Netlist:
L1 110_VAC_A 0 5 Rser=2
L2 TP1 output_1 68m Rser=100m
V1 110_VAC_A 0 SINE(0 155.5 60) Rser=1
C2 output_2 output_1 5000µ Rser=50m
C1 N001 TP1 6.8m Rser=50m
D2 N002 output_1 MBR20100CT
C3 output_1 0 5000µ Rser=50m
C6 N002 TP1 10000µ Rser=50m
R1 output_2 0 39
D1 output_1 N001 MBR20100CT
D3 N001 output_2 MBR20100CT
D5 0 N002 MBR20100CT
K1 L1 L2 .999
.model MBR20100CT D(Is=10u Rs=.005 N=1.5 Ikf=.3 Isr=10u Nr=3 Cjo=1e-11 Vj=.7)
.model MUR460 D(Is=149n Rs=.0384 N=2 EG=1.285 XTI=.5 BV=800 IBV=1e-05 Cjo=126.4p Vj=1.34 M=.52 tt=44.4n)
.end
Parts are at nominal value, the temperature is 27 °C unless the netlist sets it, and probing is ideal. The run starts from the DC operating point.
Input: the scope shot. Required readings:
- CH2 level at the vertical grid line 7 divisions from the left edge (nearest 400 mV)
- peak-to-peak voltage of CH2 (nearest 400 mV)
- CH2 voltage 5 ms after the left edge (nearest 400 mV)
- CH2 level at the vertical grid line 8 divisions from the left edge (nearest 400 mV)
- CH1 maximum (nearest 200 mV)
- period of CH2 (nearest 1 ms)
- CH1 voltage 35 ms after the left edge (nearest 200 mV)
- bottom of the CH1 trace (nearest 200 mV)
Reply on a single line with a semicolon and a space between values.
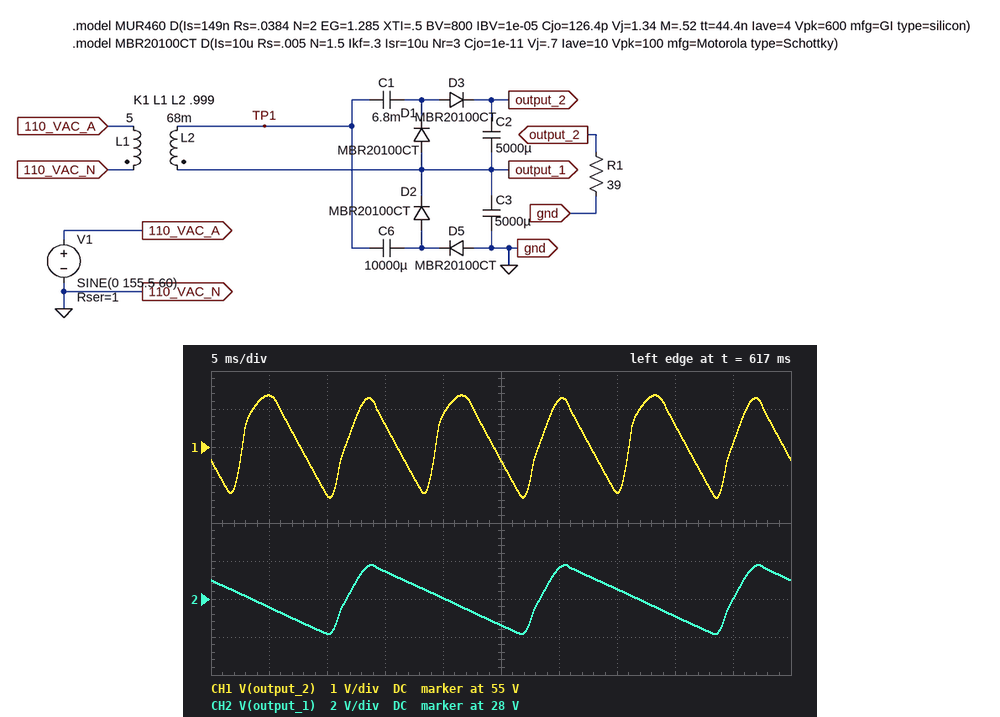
28.4 V; 3.6 V; 27.6 V; 27.2 V; 56.4 V; 17 ms; 53.8 V; 53.6 V
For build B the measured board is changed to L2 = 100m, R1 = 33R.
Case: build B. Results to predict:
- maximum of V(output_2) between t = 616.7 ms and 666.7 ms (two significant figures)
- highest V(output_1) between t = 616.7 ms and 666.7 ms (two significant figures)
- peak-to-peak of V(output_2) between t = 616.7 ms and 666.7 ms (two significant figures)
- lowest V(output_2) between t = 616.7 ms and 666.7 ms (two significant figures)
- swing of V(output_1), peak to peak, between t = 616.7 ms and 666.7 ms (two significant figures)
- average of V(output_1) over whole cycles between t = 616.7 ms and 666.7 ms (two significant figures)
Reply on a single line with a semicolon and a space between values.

66 V; 35 V; 3.5 V; 63 V; 4.9 V; 33 V
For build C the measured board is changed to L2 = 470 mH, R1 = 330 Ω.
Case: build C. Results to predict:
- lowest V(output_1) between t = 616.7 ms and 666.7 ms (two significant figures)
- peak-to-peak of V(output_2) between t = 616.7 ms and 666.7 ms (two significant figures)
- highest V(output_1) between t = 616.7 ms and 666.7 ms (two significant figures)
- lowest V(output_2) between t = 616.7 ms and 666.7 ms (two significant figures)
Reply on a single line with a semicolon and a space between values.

82 V; 1.1 V; 83 V; 160 V
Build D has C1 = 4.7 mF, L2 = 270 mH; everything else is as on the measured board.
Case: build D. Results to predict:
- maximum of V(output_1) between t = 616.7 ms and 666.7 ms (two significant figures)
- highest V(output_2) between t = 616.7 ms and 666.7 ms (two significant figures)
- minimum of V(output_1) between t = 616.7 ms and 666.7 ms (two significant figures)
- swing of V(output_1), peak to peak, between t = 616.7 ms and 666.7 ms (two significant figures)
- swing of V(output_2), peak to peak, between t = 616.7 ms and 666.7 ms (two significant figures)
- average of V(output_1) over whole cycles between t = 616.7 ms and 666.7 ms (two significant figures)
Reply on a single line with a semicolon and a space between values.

56 V; 100 V; 50 V; 6.2 V; 4.5 V; 53 V
